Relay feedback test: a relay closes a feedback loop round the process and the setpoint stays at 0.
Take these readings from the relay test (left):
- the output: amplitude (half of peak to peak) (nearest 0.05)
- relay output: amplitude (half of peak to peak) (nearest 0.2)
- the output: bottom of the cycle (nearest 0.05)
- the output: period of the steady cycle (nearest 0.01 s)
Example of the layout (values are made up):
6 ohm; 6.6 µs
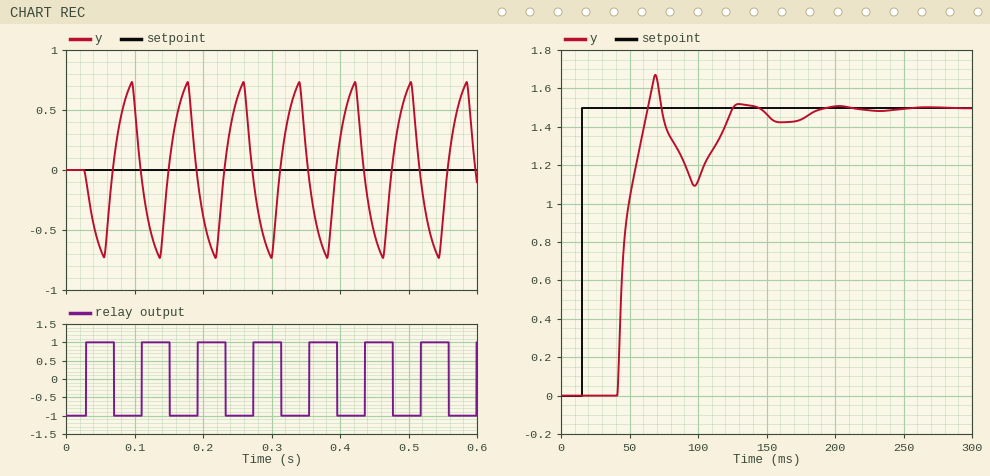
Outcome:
0.75; 1.0; -0.75; 0.08 s
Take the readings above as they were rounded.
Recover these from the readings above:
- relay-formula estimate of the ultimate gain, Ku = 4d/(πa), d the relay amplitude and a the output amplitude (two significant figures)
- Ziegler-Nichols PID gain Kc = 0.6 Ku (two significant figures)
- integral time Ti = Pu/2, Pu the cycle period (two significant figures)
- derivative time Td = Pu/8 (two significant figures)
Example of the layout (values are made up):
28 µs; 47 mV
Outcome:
1.7; 1.0; 0.040 s; 0.010 s
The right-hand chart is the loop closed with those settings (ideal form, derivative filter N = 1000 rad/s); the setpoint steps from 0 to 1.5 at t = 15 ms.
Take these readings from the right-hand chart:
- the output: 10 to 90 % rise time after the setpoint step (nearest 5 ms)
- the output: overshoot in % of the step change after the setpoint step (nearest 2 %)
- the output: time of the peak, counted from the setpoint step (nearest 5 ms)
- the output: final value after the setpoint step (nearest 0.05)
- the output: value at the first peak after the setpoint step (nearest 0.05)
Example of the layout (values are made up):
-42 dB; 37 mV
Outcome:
15 ms; 12 %; 55 ms; 1.50; 1.65
